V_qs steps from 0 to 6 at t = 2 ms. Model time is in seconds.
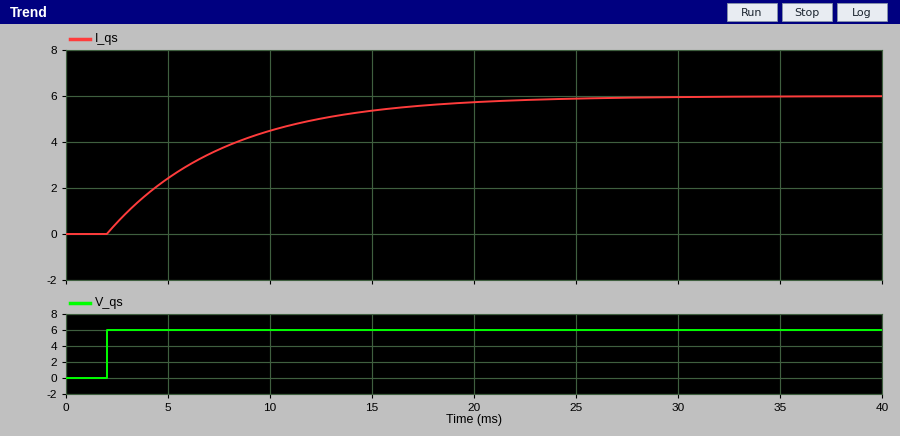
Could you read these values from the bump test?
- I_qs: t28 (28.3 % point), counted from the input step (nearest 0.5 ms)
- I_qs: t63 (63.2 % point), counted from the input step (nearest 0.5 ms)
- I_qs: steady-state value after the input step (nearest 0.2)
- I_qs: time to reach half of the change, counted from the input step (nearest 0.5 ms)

2.0 ms
6.0 ms
6.0
4.0 ms
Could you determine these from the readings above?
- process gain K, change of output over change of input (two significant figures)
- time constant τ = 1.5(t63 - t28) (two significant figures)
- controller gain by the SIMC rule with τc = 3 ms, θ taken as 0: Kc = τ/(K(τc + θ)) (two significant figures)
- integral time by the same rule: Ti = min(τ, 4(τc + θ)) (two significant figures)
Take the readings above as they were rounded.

1.0
6.0 ms
2.0
6.0 ms
